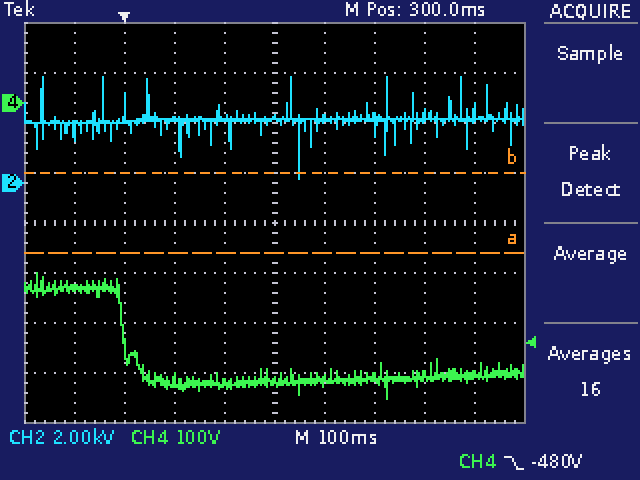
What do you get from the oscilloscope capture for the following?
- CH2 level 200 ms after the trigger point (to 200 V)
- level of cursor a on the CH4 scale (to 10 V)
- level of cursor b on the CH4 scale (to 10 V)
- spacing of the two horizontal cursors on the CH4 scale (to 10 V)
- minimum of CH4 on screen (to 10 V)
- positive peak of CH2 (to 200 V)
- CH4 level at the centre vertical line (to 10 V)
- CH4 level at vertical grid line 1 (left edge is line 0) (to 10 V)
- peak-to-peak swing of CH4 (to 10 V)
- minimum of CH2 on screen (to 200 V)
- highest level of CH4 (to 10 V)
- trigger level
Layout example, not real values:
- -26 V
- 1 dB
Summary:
- 2.6 kV
- -300 V
- -140 V
- 160 V
- -590 V
- 4.2 kV
- -560 V
- -370 V
- 250 V
- 200 V
- -340 V
- -480 V
